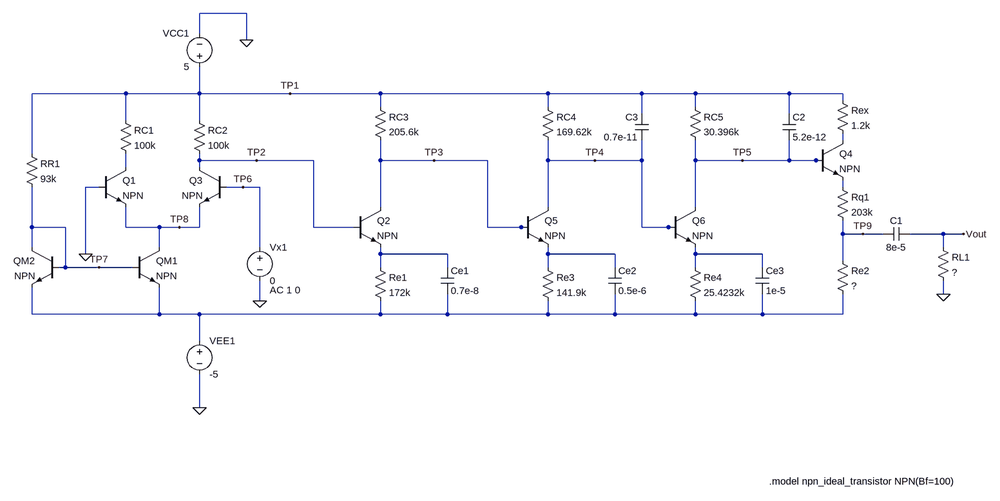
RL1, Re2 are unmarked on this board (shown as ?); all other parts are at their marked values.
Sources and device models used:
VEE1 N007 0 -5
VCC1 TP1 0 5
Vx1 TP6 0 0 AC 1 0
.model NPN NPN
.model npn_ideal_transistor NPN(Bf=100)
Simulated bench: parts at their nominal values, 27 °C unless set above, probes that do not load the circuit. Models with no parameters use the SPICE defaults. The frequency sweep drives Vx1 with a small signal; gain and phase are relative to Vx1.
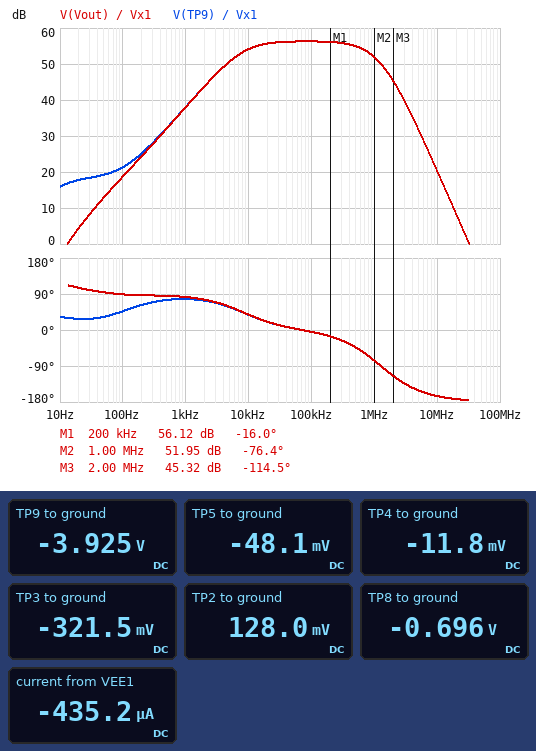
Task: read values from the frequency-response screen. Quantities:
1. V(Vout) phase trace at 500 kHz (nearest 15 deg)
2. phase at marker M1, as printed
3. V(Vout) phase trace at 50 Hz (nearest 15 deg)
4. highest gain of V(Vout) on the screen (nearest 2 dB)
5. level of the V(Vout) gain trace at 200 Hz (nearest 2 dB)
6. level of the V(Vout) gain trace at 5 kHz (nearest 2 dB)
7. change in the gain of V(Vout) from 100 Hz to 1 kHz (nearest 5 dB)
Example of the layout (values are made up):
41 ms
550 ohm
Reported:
-45 deg
-16.0 deg
90 deg
56 dB
24 dB
50 dB
20 dB
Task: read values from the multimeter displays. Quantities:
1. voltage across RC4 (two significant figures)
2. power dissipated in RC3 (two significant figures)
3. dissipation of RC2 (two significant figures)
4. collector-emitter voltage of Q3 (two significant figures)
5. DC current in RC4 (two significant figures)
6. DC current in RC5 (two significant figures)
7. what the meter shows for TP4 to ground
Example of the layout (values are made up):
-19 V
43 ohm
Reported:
5.0 V
140 µW
240 µW
820 mV
30 µA
170 µA
-11.8 mV
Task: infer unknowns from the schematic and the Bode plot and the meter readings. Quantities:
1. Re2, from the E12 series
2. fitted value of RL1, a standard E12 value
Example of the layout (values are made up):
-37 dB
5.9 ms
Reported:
68 kΩ
22 Ω
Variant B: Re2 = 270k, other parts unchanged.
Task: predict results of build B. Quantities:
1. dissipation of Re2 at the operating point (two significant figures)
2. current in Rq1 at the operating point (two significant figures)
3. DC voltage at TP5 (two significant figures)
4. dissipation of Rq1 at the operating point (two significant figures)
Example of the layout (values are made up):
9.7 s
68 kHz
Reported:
22 µW
9.1 µA
-46 mV
17 µW
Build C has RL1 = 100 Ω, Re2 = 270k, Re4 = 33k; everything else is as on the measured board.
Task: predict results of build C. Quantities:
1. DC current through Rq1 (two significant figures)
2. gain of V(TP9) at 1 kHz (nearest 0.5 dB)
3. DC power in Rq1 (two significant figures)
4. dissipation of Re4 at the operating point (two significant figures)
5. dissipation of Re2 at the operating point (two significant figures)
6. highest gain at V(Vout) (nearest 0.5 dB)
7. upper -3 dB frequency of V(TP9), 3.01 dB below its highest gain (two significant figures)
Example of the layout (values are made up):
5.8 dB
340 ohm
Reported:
11 µA
51.0 dB
26 µW
570 µW
35 µW
69.0 dB
740 kHz
